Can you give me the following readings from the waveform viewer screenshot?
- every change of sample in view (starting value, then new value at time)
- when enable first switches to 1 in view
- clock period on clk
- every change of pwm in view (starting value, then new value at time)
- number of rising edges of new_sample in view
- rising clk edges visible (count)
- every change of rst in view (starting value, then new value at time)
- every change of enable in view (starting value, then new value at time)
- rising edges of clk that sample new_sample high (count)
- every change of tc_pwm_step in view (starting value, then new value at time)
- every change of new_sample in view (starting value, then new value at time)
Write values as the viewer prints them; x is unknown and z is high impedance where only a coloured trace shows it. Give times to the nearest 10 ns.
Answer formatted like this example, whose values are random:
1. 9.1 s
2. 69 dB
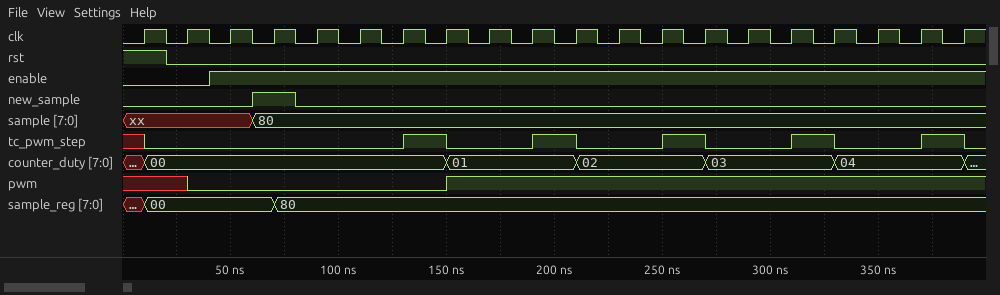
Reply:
1. xx, 80 at 60 ns
2. 40 ns
3. 20 ns
4. x, 0 at 30 ns, 1 at 150 ns
5. 1
6. 20
7. 1, 0 at 20 ns
8. 0, 1 at 40 ns
9. 1
10. x, 0 at 10 ns, 1 at 130 ns, 0 at 150 ns, 1 at 190 ns, 0 at 210 ns, 1 at 250 ns, 0 at 270 ns, 1 at 310 ns, 0 at 330 ns, 1 at 370 ns, 0 at 390 ns
11. 0, 1 at 60 ns, 0 at 80 ns
